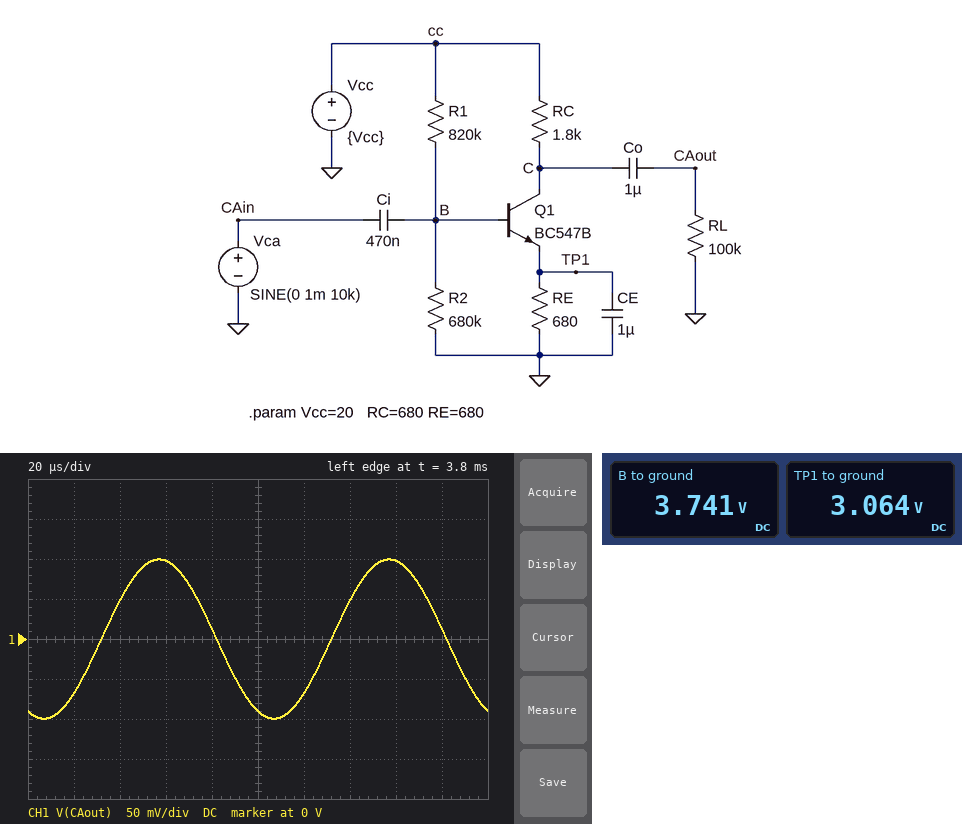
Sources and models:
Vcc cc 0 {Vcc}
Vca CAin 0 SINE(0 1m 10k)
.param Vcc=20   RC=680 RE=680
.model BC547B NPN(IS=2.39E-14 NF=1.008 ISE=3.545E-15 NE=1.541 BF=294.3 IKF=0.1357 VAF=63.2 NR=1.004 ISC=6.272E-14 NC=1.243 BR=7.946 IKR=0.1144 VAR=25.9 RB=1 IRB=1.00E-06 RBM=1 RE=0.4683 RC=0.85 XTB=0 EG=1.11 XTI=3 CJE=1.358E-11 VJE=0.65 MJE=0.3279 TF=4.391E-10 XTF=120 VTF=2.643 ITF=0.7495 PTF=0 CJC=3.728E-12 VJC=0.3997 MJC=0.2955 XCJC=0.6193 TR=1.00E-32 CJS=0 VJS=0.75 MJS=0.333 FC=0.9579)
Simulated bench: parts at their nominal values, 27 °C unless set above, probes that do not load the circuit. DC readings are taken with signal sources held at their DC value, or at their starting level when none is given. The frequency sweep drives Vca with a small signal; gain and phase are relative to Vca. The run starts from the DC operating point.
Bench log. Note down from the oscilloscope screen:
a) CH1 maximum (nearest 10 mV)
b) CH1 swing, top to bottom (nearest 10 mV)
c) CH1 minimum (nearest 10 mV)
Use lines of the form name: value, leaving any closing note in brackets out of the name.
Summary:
CH1 maximum: 100 mV
CH1 swing, top to bottom: 200 mV
CH1 minimum: -100 mV
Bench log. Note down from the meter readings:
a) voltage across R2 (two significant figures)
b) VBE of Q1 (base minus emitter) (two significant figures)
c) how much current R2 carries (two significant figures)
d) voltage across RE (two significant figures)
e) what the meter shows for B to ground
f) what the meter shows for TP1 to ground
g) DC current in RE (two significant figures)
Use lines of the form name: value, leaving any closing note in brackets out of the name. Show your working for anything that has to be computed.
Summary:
voltage across R2: 3.741 V = 3.7 V
VBE of Q1 (base minus emitter): 3.741 V - 3.064 V = 680 mV
how much current R2 carries: (3.741 V) / 680 kΩ = 5.5 µA
voltage across RE: 3.064 V = 3.1 V
what the meter shows for B to ground: 3.741 V
what the meter shows for TP1 to ground: 3.064 V
DC current in RE: (3.064 V) / 680 Ω = 4.5 mA
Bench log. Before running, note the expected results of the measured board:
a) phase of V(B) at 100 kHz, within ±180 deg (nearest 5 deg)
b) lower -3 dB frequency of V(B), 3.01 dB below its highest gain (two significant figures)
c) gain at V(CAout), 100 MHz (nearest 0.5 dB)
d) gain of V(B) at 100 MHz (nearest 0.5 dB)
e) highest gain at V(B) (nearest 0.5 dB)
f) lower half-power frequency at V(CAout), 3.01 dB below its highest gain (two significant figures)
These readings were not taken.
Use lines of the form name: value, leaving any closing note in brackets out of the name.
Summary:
phase of V(B) at 100 kHz, within ±180 deg: 0 deg
lower -3 dB frequency of V(B), 3.01 dB below its highest gain: 2.8 Hz
gain at V(CAout), 100 MHz: 42.0 dB
gain of V(B) at 100 MHz: 0 dB
highest gain at V(B): 0 dB
lower half-power frequency at V(CAout), 3.01 dB below its highest gain: 23 kHz
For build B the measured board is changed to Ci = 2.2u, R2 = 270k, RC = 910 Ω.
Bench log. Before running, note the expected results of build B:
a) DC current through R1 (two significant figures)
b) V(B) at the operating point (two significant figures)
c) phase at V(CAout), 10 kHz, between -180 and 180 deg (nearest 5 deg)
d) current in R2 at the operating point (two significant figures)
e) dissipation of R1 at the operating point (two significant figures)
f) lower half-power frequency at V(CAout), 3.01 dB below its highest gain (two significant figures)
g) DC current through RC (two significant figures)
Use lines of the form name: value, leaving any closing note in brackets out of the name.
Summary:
DC current through R1: 21 µA
V(B) at the operating point: 3.0 V
phase at V(CAout), 10 kHz, between -180 and 180 deg: -120 deg
current in R2 at the operating point: 11 µA
dissipation of R1 at the operating point: 350 µW
lower half-power frequency at V(CAout), 3.01 dB below its highest gain: 19 kHz
DC current through RC: 3.4 mA
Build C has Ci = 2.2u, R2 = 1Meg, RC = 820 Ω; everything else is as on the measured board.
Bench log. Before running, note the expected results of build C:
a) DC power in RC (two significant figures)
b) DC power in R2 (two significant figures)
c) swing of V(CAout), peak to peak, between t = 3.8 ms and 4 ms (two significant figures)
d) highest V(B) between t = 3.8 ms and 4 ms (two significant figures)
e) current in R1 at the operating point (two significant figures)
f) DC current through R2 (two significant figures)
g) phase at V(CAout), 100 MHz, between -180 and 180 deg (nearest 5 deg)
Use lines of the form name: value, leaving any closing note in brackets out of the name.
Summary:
DC power in RC: 21 mW
DC power in R2: 17 µW
swing of V(CAout), peak to peak, between t = 3.8 ms and 4 ms: 94 mV
highest V(B) between t = 3.8 ms and 4 ms: 4.1 V
current in R1 at the operating point: 19 µA
DC current through R2: 4.1 µA
phase at V(CAout), 100 MHz, between -180 and 180 deg: 135 deg
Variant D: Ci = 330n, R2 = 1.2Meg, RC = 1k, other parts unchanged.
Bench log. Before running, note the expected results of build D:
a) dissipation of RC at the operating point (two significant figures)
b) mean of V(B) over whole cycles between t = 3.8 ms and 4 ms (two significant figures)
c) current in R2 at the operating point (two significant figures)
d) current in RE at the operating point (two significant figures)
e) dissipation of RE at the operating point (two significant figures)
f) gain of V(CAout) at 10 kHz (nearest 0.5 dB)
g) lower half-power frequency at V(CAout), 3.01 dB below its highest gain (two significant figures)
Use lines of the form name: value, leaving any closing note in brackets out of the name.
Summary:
dissipation of RC at the operating point: 26 mW
mean of V(B) over whole cycles between t = 3.8 ms and 4 ms: 4.2 V
current in R2 at the operating point: 3.5 µA
current in RE at the operating point: 5.1 mA
dissipation of RE at the operating point: 18 mW
gain of V(CAout) at 10 kHz: 35.0 dB
lower half-power frequency at V(CAout), 3.01 dB below its highest gain: 27 kHz
